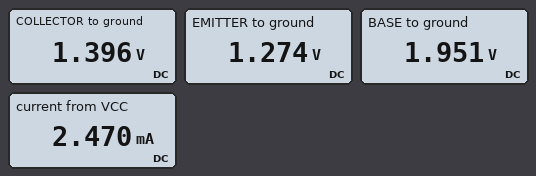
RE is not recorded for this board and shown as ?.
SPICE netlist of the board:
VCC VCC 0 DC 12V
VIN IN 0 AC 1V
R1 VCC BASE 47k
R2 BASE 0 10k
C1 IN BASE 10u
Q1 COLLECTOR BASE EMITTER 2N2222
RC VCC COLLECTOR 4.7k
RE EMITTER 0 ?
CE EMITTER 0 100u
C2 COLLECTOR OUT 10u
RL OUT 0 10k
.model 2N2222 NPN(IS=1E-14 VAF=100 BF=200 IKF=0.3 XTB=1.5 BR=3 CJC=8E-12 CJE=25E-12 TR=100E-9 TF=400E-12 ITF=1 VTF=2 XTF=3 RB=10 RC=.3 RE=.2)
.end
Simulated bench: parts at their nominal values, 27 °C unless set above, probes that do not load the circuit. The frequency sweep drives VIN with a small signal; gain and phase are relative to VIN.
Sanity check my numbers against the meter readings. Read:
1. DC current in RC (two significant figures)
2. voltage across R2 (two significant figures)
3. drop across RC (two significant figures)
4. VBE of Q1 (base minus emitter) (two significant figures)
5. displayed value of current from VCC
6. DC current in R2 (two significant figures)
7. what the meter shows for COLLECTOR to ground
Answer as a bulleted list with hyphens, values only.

- 2.3 mA
- 2.0 V
- 11 V
- 680 mV
- 2.470 mA
- 200 µA
- 1.396 V
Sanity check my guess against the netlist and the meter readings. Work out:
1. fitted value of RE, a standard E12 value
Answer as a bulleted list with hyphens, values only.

- 560 Ω
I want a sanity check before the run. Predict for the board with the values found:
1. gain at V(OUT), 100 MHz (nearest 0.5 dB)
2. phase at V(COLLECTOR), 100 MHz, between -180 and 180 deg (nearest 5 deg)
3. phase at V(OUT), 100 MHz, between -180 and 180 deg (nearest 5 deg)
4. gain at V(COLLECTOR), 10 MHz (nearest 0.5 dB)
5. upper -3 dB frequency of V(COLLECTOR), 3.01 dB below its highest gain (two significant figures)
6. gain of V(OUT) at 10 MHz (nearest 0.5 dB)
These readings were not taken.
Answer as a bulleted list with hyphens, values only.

- -1.0 dB
- 40 deg
- 40 deg
- 17.5 dB
- 1.5 MHz
- 17.5 dB
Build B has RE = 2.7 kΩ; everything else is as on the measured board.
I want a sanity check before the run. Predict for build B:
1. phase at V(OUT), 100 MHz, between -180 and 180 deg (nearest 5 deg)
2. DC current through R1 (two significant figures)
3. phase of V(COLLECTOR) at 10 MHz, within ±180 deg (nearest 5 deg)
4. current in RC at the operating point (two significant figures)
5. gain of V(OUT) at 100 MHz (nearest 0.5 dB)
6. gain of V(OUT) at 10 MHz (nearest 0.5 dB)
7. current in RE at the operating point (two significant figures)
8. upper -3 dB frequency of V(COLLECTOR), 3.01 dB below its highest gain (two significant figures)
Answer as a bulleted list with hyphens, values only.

- 75 deg
- 210 µA
- 135 deg
- 530 µA
- 17.0 dB
- 33.5 dB
- 540 µA
- 11 MHz
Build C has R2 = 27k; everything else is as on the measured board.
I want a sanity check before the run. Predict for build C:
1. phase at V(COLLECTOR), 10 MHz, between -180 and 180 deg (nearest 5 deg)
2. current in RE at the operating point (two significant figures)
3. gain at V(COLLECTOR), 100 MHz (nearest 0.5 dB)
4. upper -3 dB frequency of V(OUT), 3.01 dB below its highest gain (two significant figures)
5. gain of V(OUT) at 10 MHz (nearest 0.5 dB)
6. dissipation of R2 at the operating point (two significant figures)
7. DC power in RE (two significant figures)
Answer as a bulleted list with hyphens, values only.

- 50 deg
- 2.4 mA
- -6.5 dB
- 1.3 MHz
- -3.5 dB
- 150 µW
- 3.2 mW
